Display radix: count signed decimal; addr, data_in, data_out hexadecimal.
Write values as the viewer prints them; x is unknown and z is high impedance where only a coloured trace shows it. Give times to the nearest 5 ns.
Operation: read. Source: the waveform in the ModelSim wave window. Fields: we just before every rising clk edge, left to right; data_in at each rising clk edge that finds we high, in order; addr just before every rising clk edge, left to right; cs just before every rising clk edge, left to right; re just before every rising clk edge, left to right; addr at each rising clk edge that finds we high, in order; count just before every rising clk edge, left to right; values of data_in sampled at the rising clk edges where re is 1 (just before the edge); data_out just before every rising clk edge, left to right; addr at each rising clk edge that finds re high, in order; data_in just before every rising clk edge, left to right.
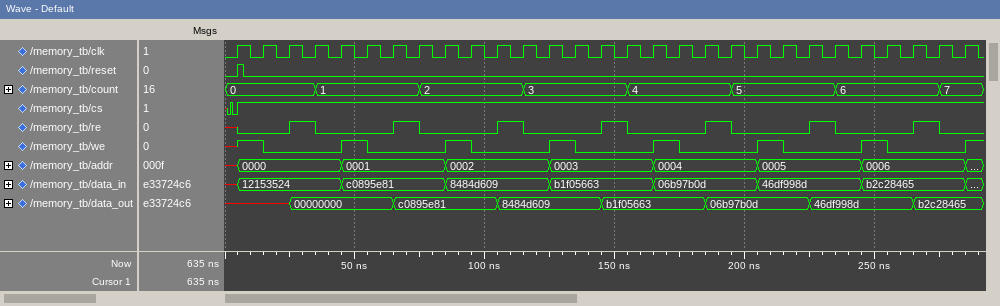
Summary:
x 1 0 0 0 1 0 0 0 1 0 0 0 1 0 0 0 1 0 0 0 1 0 0 0 1 0 0 0
12153524, c0895e81, 8484d609, b1f05663, 06b97b0d, 46df998d, b2c28465
x, 0000, 0000, 0000, 0000, 0001, 0001, 0001, 0001, 0002, 0002, 0002, 0002, 0003, 0003, 0003, 0003, 0004, 0004, 0004, 0004, 0005, 0005, 0005, 0005, 0006, 0006, 0006, 0006
0 1 1 1 1 1 1 1 1 1 1 1 1 1 1 1 1 1 1 1 1 1 1 1 1 1 1 1 1
x 0 0 1 0 0 0 1 0 0 0 1 0 0 0 1 0 0 0 1 0 0 0 1 0 0 0 1 0
0000, 0001, 0002, 0003, 0004, 0005, 0006
0, 0, 0, 0, 1, 1, 1, 1, 2, 2, 2, 2, 3, 3, 3, 3, 4, 4, 4, 4, 5, 5, 5, 5, 6, 6, 6, 6, 7
12153524, c0895e81, 8484d609, b1f05663, 06b97b0d, 46df998d, b2c28465
x, x, x, 00000000, 00000000, 00000000, 00000000, c0895e81, c0895e81, c0895e81, c0895e81, 8484d609, 8484d609, 8484d609, 8484d609, b1f05663, b1f05663, b1f05663, b1f05663, 06b97b0d, 06b97b0d, 06b97b0d, 06b97b0d, 46df998d, 46df998d, 46df998d, 46df998d, b2c28465, b2c28465
0000, 0001, 0002, 0003, 0004, 0005, 0006
x, 12153524, 12153524, 12153524, 12153524, c0895e81, c0895e81, c0895e81, c0895e81, 8484d609, 8484d609, 8484d609, 8484d609, b1f05663, b1f05663, b1f05663, b1f05663, 06b97b0d, 06b97b0d, 06b97b0d, 06b97b0d, 46df998d, 46df998d, 46df998d, 46df998d, b2c28465, b2c28465, b2c28465, b2c28465
